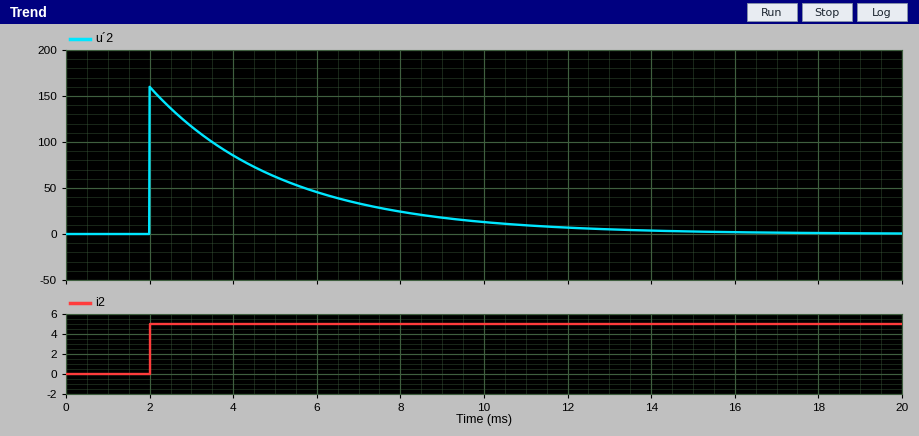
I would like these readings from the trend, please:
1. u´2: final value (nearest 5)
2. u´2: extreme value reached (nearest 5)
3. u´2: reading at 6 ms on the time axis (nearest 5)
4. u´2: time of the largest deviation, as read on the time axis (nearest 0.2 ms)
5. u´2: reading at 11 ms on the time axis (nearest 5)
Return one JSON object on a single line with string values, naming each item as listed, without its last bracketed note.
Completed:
{"u´2: final value": "0", "u´2: extreme value reached": "160", "u´2: reading at 6 ms on the time axis": "45", "u´2: time of the largest deviation, as read on the time axis": "2.0 ms", "u´2: reading at 11 ms on the time axis": "10"}
